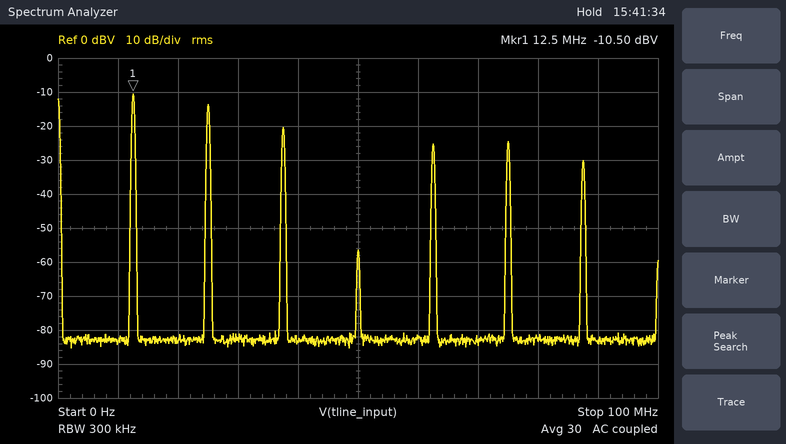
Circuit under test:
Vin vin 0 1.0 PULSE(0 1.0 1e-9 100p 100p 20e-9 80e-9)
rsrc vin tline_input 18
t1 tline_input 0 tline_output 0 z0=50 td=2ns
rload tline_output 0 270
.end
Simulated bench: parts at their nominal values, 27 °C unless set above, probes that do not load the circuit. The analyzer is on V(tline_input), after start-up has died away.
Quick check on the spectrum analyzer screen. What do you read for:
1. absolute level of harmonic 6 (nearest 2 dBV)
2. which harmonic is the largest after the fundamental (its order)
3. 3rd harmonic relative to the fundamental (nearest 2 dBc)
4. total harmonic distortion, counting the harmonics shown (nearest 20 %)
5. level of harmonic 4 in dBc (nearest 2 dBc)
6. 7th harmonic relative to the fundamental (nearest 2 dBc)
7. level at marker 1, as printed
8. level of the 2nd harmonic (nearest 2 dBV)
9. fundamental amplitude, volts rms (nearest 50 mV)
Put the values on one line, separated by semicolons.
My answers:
-24 dBV; 2; -10 dBc; 80 %; -46 dBc; -20 dBc; -10.50 dBV; -14 dBV; 300 mV
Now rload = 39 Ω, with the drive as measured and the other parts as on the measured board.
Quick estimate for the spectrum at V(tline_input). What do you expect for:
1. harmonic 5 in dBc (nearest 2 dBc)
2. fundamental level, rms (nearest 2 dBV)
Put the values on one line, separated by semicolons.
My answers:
-14 dBc; -14 dBV
